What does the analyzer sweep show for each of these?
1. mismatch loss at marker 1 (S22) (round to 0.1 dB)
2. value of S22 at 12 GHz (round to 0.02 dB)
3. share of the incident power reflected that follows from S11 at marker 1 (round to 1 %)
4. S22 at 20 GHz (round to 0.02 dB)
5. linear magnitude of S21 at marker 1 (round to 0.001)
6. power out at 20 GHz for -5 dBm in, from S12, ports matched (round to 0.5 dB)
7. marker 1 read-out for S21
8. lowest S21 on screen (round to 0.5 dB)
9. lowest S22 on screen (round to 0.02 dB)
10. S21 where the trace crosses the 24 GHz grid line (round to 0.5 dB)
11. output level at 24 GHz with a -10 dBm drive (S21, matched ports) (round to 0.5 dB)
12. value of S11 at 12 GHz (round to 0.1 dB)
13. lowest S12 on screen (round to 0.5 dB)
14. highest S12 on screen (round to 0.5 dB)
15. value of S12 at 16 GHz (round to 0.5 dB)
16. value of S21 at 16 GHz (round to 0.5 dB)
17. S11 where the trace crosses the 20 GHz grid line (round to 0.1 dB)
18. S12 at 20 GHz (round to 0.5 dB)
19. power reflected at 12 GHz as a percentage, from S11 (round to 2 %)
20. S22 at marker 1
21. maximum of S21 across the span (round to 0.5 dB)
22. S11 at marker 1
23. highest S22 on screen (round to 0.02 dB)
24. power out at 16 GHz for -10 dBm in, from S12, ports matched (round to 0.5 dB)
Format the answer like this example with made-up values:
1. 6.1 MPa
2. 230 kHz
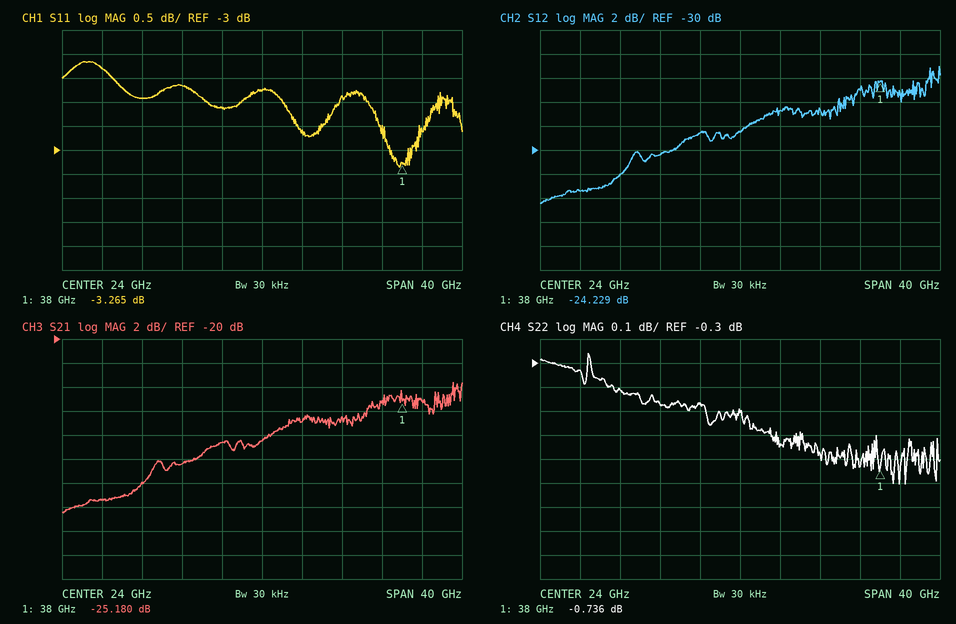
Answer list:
1. 8.1 dB
2. -0.42 dB
3. 47 %
4. -0.46 dB
5. 0.055
6. -33.5 dBm
7. -25.180 dB
8. -34.5 dB
9. -0.80 dB
10. -28.5 dB
11. -38.5 dBm
12. -1.9 dB
13. -34.5 dB
14. -23.0 dB
15. -30.5 dB
16. -30.5 dB
17. -2.1 dB
18. -28.5 dB
19. 64 %
20. -0.736 dB
21. -23.5 dB
22. -3.265 dB
23. -0.26 dB
24. -40.5 dBm
